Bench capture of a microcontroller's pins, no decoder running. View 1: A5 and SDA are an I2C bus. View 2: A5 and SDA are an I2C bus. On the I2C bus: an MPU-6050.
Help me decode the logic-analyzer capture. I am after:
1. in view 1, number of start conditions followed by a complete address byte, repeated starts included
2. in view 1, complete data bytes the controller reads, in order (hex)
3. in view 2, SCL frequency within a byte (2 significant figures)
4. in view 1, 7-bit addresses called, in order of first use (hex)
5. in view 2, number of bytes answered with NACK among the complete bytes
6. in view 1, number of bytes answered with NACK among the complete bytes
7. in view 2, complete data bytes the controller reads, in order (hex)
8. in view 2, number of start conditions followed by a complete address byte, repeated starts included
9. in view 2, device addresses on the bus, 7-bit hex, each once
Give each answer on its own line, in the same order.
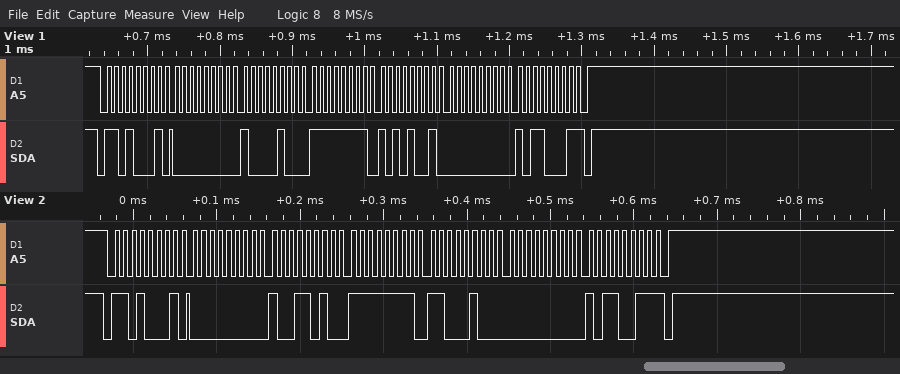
1
00 84 FF A9 00 B1
100 kHz
0x68
1
1
00 9A FF C4 00 B3
1
0x68
